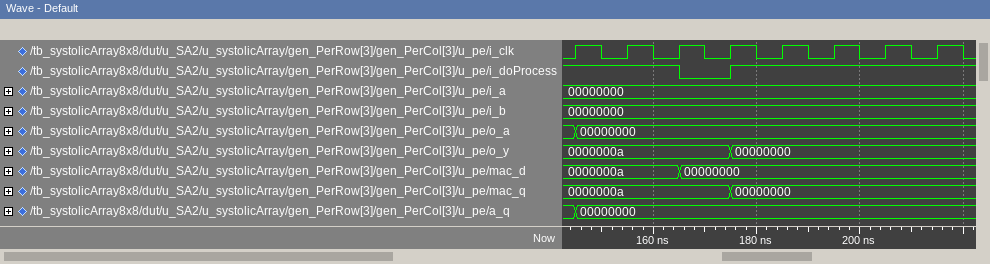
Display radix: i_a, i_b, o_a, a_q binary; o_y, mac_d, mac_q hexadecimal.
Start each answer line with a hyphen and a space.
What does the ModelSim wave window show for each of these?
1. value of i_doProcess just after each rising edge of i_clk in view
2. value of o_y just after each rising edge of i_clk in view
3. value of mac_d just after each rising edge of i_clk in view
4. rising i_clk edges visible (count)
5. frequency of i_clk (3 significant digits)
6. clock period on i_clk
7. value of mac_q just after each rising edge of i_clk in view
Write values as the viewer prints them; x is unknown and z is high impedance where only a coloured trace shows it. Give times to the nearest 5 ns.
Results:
- 1 1 0 1 1 1 1 1
- 0000000a, 0000000a, 0000000a, 00000000, 00000000, 00000000, 00000000, 00000000
- 0000000a, 0000000a, 00000000, 00000000, 00000000, 00000000, 00000000, 00000000
- 8
- 100 MHz
- 10 ns
- 0000000a, 0000000a, 0000000a, 00000000, 00000000, 00000000, 00000000, 00000000
